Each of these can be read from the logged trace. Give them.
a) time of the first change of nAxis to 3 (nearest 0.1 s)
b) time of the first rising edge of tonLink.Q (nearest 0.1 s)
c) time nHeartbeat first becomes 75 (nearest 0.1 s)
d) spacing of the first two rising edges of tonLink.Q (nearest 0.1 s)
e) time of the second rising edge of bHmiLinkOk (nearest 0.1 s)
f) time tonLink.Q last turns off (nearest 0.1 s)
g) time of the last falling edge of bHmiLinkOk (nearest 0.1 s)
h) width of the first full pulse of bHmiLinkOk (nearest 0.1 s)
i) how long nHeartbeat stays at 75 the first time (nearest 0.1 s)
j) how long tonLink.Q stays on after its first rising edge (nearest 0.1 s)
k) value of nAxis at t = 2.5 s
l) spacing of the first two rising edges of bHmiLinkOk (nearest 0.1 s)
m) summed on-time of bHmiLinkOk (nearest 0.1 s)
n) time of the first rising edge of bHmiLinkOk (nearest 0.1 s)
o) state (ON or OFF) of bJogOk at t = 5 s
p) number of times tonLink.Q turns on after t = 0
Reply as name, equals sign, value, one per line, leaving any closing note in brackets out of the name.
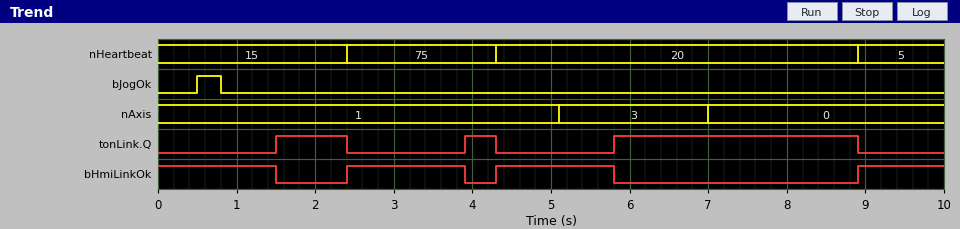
time of the first change of nAxis to 3 = 5.1 s
time of the first rising edge of tonLink.Q = 1.5 s
time nHeartbeat first becomes 75 = 2.4 s
spacing of the first two rising edges of tonLink.Q = 2.4 s
time of the second rising edge of bHmiLinkOk = 4.3 s
time tonLink.Q last turns off = 8.9 s
time of the last falling edge of bHmiLinkOk = 5.8 s
width of the first full pulse of bHmiLinkOk = 1.5 s
how long nHeartbeat stays at 75 the first time = 1.9 s
how long tonLink.Q stays on after its first rising edge = 0.9 s
value of nAxis at t = 2.5 s = 1
spacing of the first two rising edges of bHmiLinkOk = 1.9 s
summed on-time of bHmiLinkOk = 5.6 s
time of the first rising edge of bHmiLinkOk = 2.4 s
state (ON or OFF) of bJogOk at t = 5 s = OFF
number of times tonLink.Q turns on after t = 0 = 3
